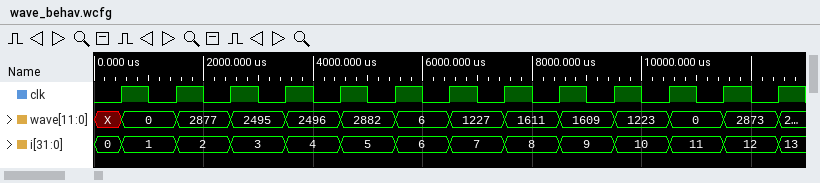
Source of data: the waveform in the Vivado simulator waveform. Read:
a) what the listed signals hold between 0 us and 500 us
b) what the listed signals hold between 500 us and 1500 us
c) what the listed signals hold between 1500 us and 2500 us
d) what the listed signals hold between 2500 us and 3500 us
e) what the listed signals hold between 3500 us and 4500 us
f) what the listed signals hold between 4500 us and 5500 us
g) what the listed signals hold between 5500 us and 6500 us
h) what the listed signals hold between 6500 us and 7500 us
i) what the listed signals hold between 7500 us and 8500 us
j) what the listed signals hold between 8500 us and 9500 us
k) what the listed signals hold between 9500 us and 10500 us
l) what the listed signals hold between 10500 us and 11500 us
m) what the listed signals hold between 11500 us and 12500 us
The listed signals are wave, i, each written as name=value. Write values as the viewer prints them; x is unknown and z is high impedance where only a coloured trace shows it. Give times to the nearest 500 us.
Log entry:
wave=X, i=0
wave=0, i=1
wave=2877, i=2
wave=2495, i=3
wave=2496, i=4
wave=2882, i=5
wave=6, i=6
wave=1227, i=7
wave=1611, i=8
wave=1609, i=9
wave=1223, i=10
wave=0, i=11
wave=2873, i=12
